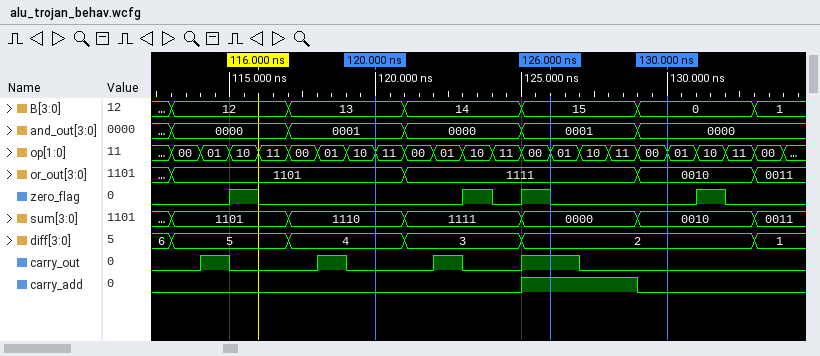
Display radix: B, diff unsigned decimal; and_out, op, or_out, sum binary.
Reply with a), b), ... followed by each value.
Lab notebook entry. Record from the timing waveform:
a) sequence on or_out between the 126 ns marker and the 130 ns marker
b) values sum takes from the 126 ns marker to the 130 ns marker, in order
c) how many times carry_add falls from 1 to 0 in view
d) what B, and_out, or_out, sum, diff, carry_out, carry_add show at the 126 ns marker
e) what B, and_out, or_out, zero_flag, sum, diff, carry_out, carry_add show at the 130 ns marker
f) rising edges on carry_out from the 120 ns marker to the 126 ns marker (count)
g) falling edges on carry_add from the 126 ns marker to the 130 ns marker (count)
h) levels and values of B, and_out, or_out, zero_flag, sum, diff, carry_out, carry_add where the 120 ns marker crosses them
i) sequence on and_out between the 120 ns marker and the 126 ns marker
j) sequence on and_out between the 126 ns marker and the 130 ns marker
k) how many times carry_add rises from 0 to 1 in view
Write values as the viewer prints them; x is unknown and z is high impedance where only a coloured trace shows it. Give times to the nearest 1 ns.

a) 1111, 0010
b) 0000, 0010
c) 1
d) B=15, and_out=0001, or_out=1111, sum=0000, diff=2, carry_out=1, carry_add=1
e) B=0, and_out=0000, or_out=0010, zero_flag=0, sum=0010, diff=2, carry_out=0, carry_add=0
f) 2
g) 1
h) B=13, and_out=0001, or_out=1101, zero_flag=0, sum=1110, diff=4, carry_out=0, carry_add=0
i) 0001, 0000, 0001
j) 0001, 0000
k) 1
